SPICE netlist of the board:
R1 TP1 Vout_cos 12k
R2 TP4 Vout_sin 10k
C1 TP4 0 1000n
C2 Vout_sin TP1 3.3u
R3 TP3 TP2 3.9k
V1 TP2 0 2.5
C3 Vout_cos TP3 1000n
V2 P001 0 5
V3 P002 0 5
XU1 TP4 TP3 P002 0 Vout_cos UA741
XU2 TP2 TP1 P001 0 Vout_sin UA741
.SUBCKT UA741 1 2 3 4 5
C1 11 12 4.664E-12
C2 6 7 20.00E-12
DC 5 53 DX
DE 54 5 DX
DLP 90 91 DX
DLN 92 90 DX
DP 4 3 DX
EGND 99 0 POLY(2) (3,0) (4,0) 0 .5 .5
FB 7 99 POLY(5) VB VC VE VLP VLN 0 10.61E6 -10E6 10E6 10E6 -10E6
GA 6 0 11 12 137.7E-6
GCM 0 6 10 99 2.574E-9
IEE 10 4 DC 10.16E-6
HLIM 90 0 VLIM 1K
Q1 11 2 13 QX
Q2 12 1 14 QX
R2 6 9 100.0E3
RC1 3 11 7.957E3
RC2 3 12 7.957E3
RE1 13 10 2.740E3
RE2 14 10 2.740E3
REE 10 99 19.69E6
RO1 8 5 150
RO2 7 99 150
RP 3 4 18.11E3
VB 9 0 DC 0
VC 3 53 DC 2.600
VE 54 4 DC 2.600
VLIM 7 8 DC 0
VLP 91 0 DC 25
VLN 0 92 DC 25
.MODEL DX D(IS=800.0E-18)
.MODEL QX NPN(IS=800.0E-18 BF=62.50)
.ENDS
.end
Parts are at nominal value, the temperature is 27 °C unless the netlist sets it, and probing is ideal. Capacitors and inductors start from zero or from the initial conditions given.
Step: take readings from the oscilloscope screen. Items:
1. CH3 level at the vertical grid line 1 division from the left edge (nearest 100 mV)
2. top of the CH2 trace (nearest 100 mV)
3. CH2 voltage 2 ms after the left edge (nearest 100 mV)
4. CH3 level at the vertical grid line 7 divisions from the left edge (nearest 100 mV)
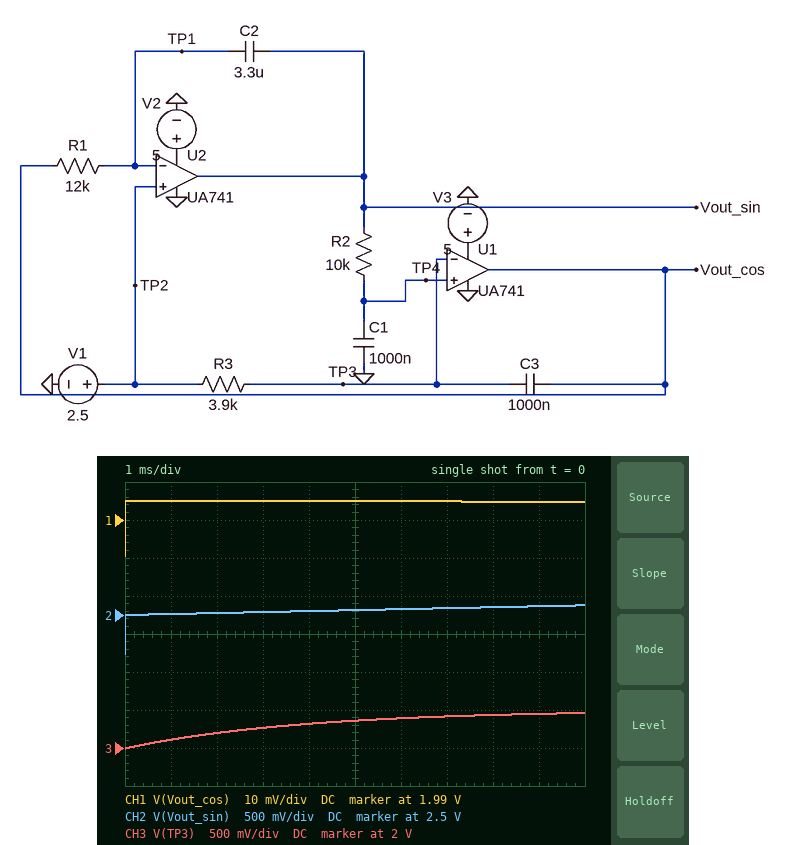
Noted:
2.1 V
2.6 V
2.5 V
2.4 V
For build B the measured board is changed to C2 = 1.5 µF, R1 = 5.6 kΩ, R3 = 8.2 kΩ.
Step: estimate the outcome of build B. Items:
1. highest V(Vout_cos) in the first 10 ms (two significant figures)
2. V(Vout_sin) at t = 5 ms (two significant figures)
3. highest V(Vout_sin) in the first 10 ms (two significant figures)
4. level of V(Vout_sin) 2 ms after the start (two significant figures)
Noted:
2.0 V
2.8 V
3.0 V
2.6 V
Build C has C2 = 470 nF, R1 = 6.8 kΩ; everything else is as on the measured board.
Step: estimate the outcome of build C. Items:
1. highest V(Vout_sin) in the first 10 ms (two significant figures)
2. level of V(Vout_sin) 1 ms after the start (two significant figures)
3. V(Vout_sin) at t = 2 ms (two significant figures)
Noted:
3.0 V
2.7 V
2.8 V
